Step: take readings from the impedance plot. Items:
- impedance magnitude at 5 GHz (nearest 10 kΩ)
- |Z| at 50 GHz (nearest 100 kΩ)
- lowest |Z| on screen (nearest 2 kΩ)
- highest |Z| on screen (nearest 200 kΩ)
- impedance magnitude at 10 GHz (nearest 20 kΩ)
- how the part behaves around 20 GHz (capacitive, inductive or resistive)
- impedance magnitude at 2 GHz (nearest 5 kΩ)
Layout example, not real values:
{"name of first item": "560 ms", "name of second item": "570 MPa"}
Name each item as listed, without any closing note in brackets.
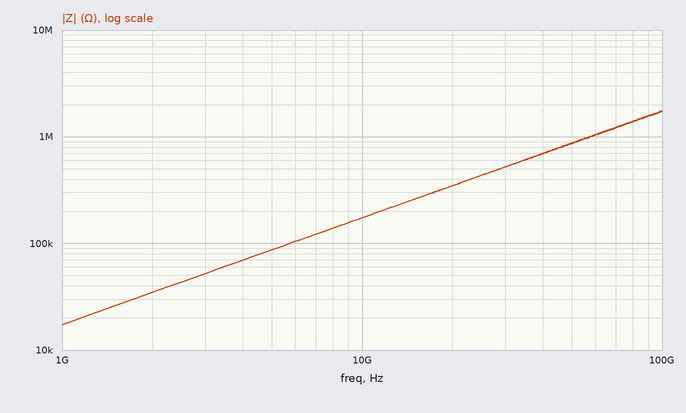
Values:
{"impedance magnitude at 5 GHz": "90 kΩ", "|Z| at 50 GHz": "900 kΩ", "lowest |Z| on screen": "18 kΩ", "highest |Z| on screen": "1.8 MΩ", "impedance magnitude at 10 GHz": "180 kΩ", "how the part behaves around 20 GHz": "inductive", "impedance magnitude at 2 GHz": "35 kΩ"}
